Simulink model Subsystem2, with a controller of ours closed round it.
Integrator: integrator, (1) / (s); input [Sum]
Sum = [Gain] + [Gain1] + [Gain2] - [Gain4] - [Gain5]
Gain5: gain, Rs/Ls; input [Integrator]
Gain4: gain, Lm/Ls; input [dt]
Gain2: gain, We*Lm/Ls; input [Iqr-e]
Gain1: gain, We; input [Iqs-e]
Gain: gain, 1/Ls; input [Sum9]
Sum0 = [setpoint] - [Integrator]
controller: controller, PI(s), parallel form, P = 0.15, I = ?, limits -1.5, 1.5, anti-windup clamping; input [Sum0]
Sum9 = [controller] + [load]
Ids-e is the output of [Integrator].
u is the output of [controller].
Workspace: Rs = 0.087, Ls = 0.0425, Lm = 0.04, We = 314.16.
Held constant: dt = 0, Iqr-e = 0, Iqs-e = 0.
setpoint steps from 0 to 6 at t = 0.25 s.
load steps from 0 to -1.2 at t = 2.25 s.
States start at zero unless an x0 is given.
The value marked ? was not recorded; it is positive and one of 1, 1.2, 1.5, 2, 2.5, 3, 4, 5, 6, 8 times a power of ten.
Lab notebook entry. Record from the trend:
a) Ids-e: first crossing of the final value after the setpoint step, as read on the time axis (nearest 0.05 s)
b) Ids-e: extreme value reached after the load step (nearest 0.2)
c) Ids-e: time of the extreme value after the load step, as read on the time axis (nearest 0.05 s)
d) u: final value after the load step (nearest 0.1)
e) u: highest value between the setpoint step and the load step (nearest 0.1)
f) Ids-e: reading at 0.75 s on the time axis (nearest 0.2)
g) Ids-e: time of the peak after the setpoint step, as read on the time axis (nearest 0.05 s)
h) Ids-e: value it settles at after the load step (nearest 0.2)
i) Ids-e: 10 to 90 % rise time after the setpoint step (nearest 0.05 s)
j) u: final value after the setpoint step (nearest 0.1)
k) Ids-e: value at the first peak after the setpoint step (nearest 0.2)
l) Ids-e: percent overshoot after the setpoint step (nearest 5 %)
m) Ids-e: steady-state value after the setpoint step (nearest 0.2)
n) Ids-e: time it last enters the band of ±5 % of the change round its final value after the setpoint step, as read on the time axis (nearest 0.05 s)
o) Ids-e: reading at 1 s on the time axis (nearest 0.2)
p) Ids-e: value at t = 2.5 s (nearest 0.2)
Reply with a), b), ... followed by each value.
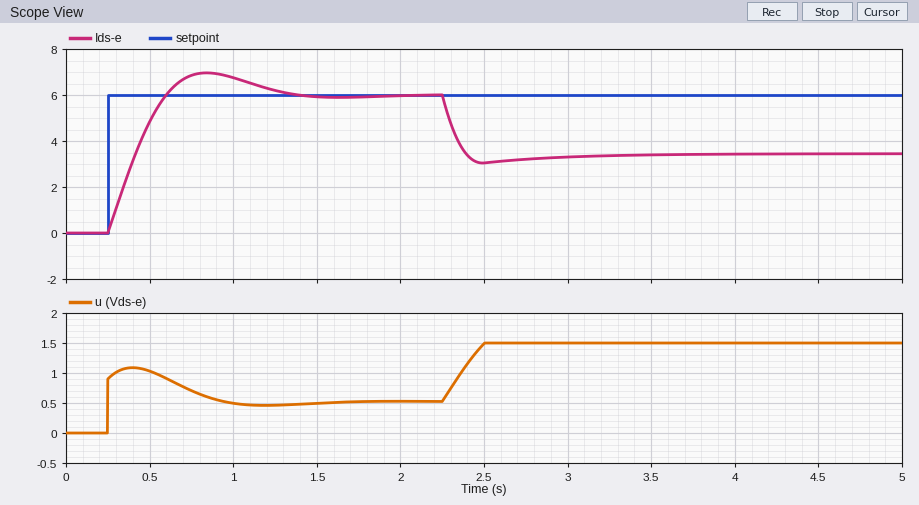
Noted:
a) 0.60 s
b) 3.0
c) 2.50 s
d) 1.5
e) 1.1
f) 6.8
g) 0.85 s
h) 3.4
i) 0.25 s
j) 0.5
k) 7.0
l) 15 %
m) 6.0
n) 1.20 s
o) 6.8
p) 3.0
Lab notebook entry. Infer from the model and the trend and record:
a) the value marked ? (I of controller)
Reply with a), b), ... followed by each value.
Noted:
a) 1
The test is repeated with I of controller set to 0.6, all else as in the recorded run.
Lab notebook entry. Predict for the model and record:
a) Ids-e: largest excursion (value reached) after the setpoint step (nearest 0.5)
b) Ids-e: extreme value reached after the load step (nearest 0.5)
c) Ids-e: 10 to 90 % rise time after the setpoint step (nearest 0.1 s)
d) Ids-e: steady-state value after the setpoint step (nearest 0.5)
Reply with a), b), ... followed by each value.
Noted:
a) 6.5
b) 2.5
c) 0.4 s
d) 6.0
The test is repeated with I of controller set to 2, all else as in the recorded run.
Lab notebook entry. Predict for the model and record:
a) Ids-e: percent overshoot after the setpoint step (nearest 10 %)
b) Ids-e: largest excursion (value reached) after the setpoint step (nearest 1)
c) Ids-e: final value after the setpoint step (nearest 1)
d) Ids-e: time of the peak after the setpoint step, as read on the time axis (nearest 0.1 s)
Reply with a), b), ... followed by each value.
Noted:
a) 30 %
b) 8
c) 6
d) 0.7 s
